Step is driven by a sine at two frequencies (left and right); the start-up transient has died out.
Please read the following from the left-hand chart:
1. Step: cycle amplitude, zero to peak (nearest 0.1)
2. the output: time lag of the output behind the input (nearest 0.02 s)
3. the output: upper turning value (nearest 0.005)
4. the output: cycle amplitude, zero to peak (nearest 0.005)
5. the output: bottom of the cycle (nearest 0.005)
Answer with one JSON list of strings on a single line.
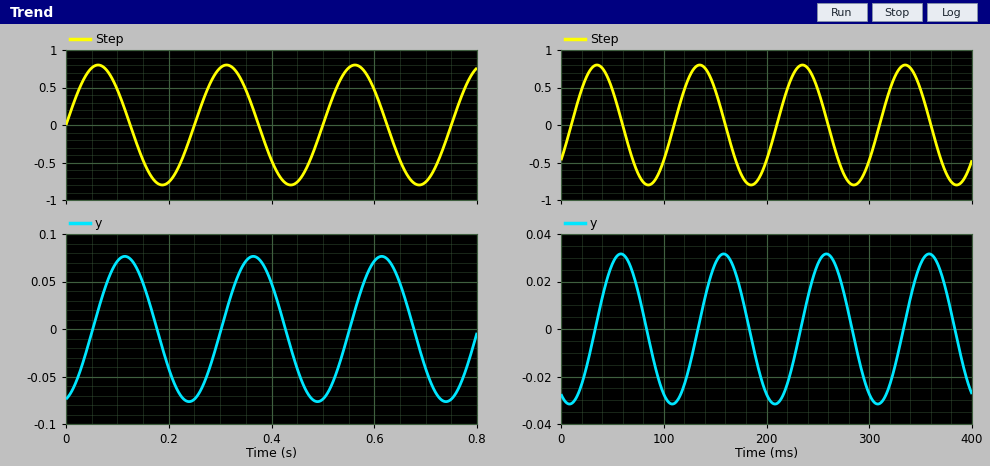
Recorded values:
["0.8", "0.06 s", "0.075", "0.075", "-0.075"]
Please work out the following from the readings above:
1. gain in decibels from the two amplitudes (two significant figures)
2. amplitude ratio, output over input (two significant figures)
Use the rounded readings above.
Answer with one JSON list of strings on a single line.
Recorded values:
["-21 dB", "0.094"]
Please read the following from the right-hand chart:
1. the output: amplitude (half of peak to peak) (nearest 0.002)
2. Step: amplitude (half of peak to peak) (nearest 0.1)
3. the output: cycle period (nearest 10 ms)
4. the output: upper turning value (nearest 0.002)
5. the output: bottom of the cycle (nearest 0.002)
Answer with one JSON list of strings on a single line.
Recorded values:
["0.032", "0.8", "100 ms", "0.032", "-0.032"]
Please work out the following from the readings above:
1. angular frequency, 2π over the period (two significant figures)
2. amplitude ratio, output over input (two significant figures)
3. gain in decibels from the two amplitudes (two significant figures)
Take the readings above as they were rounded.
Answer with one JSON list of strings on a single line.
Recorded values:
["0.063 rad/ms", "0.040", "-28 dB"]
